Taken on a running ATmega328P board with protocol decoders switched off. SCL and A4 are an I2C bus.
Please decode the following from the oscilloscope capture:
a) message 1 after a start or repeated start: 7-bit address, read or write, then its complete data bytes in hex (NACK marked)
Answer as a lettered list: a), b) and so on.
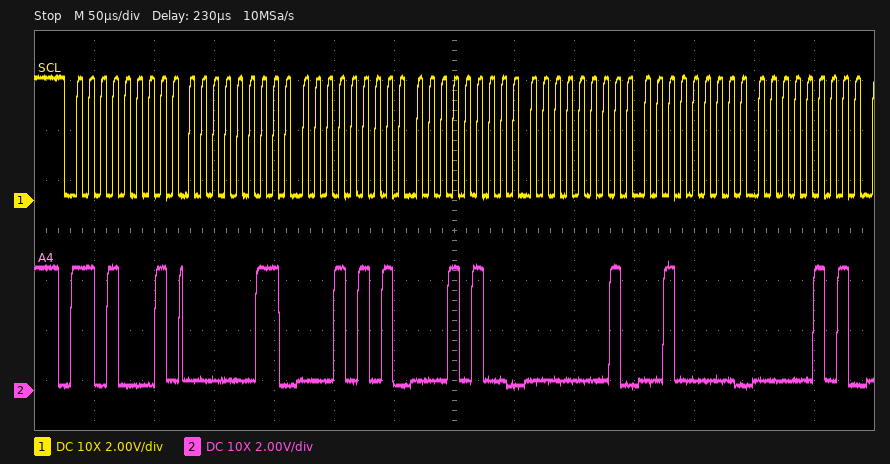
a) 0x68 read: 03 15 14 01 20 05
